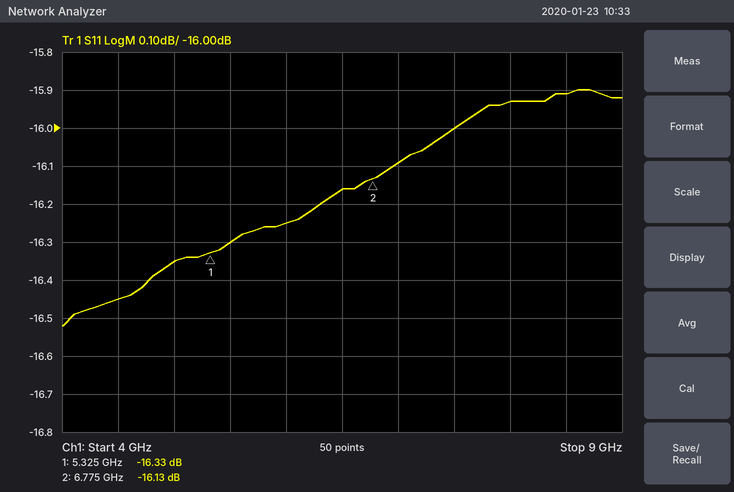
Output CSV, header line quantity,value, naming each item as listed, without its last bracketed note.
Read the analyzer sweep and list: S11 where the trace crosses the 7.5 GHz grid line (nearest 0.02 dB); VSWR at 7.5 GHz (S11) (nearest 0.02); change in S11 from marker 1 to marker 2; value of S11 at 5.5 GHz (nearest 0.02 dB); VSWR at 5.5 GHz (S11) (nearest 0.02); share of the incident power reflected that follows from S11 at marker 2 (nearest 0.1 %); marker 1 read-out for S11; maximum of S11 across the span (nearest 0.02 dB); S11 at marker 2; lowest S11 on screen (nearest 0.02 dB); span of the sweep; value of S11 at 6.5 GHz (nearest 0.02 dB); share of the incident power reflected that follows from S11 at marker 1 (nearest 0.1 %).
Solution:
quantity,value
S11 where the trace crosses the 7.5 GHz grid line,-16.00 dB
VSWR at 7.5 GHz (S11),1.38
change in S11 from marker 1 to marker 2,0.20 dB
value of S11 at 5.5 GHz,-16.30 dB
VSWR at 5.5 GHz (S11),1.36
share of the incident power reflected that follows from S11 at marker 2,2.4 %
marker 1 read-out for S11,-16.33 dB
maximum of S11 across the span,-15.90 dB
S11 at marker 2,-16.13 dB
lowest S11 on screen,-16.52 dB
span of the sweep,5 GHz
value of S11 at 6.5 GHz,-16.16 dB
share of the incident power reflected that follows from S11 at marker 1,2.3 %
